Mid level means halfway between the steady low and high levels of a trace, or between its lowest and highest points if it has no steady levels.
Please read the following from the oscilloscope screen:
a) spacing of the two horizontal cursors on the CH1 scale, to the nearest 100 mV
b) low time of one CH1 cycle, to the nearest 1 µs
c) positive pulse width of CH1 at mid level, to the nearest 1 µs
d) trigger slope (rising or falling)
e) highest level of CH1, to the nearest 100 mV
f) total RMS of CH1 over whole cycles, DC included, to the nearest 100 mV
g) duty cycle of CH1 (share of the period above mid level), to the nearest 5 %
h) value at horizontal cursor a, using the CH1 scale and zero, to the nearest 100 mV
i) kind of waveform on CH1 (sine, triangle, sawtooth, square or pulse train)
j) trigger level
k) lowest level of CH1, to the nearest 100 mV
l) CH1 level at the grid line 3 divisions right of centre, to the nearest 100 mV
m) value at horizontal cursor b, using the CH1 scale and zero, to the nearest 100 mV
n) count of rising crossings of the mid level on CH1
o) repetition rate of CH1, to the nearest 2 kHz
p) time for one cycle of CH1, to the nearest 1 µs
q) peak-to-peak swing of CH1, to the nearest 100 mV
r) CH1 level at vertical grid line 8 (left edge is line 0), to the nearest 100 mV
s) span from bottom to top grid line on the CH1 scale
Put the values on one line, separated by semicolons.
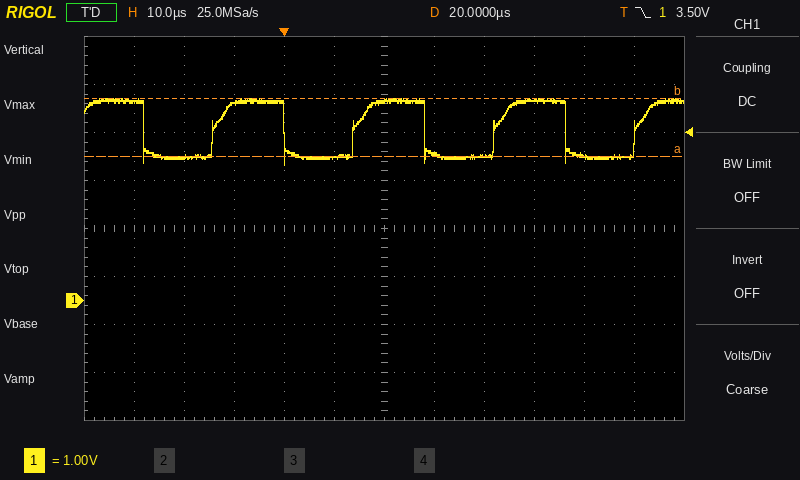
1.2 V; 14 µs; 14 µs; falling; 4.2 V; 3.6 V; 50 %; 3.0 V; square; 3.50 V; 2.8 V; 4.2 V; 4.2 V; 4; 36 kHz; 28 µs; 1.4 V; 3.0 V; 8 V
